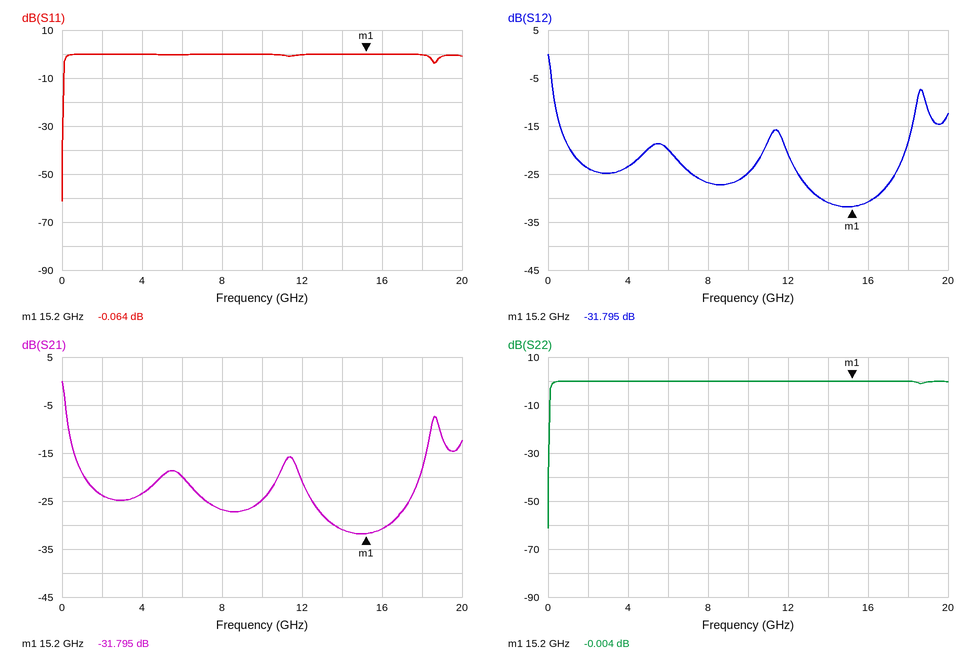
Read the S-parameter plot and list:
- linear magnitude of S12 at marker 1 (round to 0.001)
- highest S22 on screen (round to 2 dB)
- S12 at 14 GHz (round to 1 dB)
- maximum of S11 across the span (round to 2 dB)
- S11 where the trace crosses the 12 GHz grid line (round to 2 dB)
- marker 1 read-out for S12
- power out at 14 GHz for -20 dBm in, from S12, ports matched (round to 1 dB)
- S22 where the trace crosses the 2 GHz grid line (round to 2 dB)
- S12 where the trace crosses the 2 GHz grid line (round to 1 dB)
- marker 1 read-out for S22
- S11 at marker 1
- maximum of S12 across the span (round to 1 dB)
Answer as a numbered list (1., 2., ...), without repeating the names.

1. 0.026
2. 0 dB
3. -31 dB
4. 0 dB
5. 0 dB
6. -31.795 dB
7. -51 dBm
8. 0 dB
9. -24 dB
10. -0.004 dB
11. -0.064 dB
12. 0 dB
